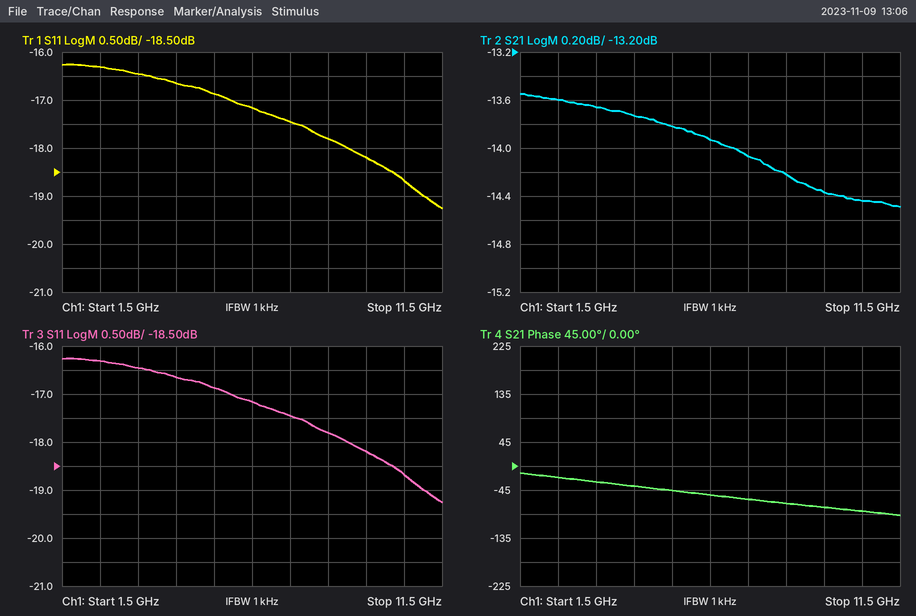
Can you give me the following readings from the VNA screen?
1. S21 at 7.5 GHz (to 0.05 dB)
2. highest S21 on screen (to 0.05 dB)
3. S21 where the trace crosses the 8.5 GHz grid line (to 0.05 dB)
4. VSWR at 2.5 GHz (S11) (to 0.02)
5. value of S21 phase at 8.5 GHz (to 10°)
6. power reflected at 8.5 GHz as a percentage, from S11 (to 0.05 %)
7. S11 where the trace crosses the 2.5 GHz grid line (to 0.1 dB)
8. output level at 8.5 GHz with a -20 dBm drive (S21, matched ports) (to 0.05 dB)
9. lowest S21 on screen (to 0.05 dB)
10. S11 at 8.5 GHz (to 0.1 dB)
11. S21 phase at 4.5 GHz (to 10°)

-14.05 dB
-13.55 dB
-14.20 dB
1.36
-70°
1.65 %
-16.3 dB
-34.20 dBm
-14.50 dB
-17.8 dB
-40°
